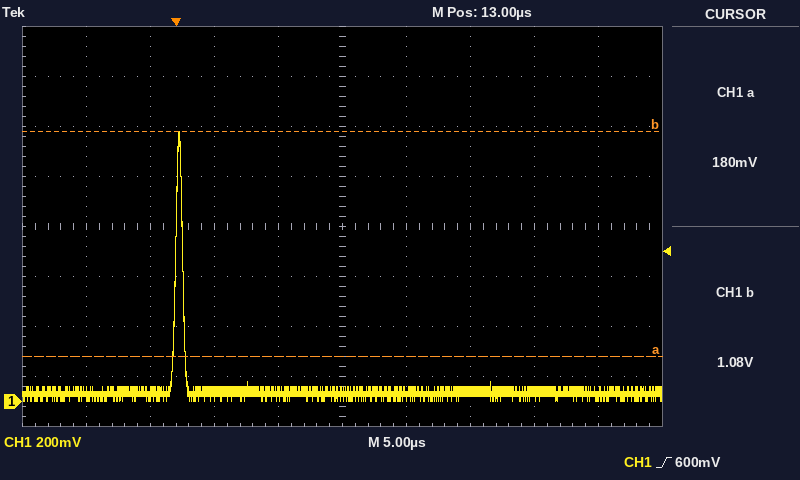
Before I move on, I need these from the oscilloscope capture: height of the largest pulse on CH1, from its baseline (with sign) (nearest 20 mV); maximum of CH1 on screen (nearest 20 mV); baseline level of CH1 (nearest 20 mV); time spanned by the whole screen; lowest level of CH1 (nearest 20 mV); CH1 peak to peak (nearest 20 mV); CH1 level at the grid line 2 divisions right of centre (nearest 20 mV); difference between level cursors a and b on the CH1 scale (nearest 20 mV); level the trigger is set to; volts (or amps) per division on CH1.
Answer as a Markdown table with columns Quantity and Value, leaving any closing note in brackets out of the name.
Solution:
| Quantity | Value |
|---|---|
| height of the largest pulse on CH1, from its baseline (with sign) | +1.04 V |
| maximum of CH1 on screen | 1.08 V |
| baseline level of CH1 | 40 mV |
| time spanned by the whole screen | 50 µs |
| lowest level of CH1 | 0 mV |
| CH1 peak to peak | 1.08 V |
| CH1 level at the grid line 2 divisions right of centre | 40 mV |
| difference between level cursors a and b on the CH1 scale | 900 mV |
| level the trigger is set to | 600 mV |
| volts (or amps) per division on CH1 | 200 mV |
